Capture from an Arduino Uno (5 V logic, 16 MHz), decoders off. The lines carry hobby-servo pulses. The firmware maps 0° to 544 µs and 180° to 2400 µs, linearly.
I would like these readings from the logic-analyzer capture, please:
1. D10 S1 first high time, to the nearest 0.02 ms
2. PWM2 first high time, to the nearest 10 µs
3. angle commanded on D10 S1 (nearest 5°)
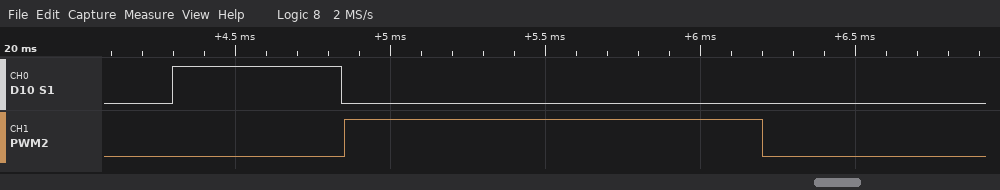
0.54 ms
1350 µs
0°
